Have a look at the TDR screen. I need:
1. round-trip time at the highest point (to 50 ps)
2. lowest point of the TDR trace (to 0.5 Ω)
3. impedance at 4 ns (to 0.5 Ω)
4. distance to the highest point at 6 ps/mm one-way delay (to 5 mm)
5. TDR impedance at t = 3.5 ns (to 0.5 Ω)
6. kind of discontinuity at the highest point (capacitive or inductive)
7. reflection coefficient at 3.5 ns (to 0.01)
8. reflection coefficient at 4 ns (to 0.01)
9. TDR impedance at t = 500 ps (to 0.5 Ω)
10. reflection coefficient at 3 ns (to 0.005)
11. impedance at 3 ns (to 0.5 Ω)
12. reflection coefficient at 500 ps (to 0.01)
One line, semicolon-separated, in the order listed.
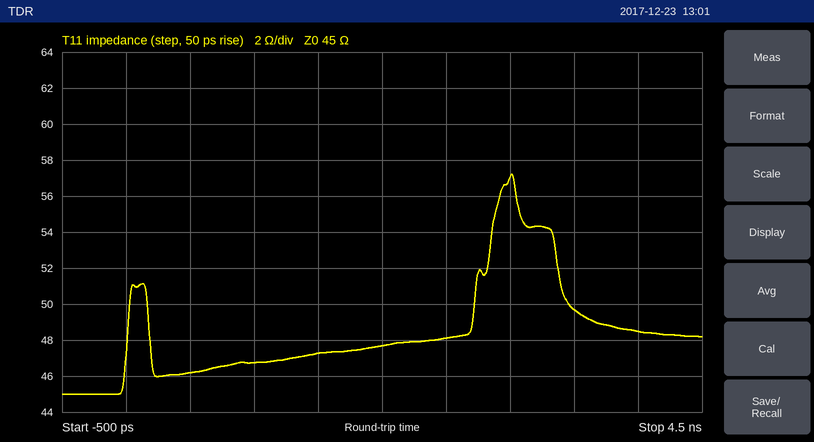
3.00 ns; 45.0 Ω; 48.5 Ω; 250 mm; 49.5 Ω; inductive; +0.05; +0.04; 46.0 Ω; +0.120; 57.0 Ω; +0.01
